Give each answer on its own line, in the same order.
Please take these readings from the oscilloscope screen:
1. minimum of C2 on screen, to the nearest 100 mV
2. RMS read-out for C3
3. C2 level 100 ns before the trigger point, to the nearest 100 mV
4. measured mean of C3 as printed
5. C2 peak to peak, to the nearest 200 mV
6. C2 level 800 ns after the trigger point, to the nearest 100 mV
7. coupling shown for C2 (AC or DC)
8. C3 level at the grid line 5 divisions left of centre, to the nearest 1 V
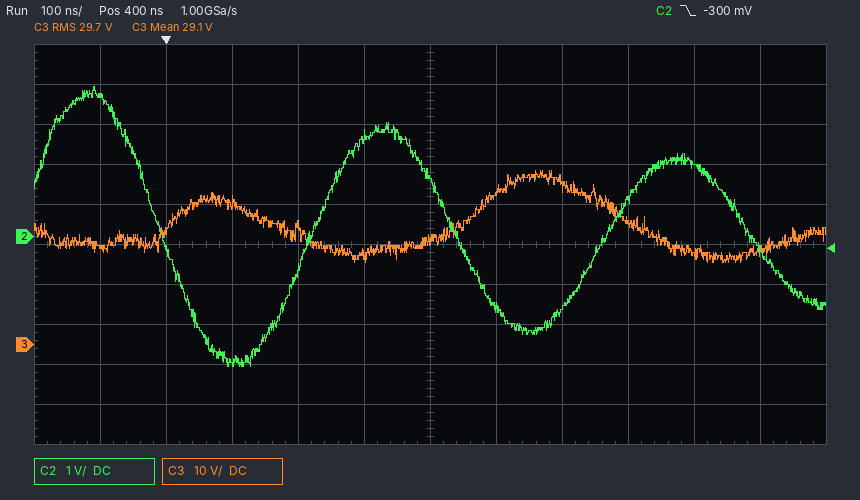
-3.2 V
29.7 V
3.5 V
29.1 V
7.0 V
1.8 V
DC
24 V
